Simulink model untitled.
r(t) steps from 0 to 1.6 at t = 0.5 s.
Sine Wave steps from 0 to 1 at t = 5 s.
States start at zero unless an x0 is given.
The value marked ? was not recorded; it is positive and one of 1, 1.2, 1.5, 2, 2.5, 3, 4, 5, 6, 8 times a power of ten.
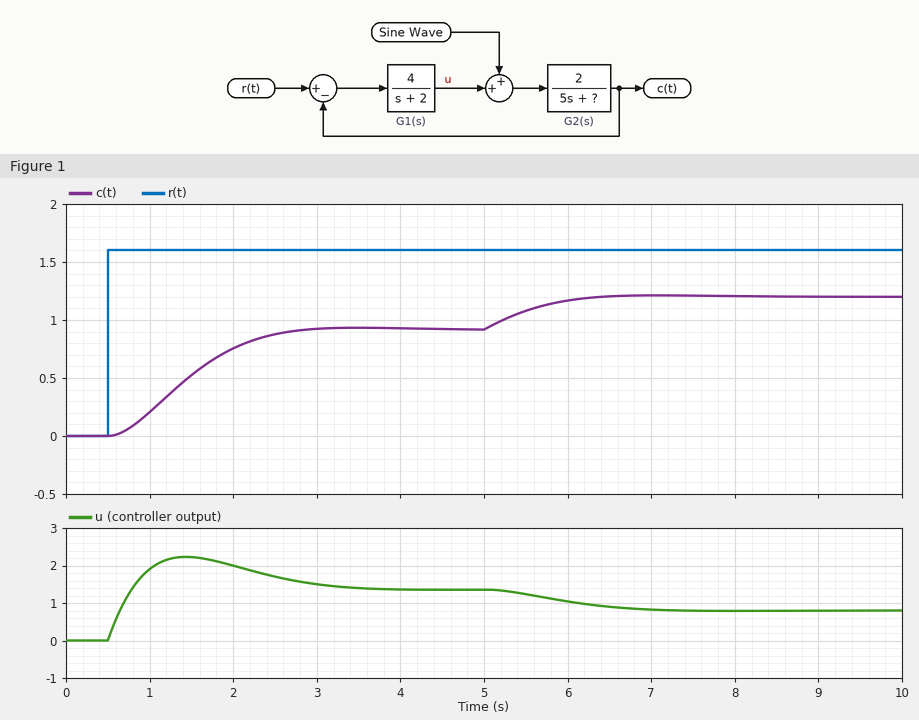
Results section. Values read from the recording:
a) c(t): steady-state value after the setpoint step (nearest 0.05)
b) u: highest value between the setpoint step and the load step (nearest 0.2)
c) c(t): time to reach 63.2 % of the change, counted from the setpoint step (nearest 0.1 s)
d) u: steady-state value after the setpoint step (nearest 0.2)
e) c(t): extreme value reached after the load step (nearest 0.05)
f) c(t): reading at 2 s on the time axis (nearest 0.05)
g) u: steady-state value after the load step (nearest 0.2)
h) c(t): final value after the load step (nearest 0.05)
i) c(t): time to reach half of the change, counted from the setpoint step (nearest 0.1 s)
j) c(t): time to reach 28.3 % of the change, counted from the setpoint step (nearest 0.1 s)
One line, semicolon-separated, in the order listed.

0.90; 2.2; 1.1 s; 1.4; 1.20; 0.75; 0.8; 1.20; 0.9 s; 0.6 s
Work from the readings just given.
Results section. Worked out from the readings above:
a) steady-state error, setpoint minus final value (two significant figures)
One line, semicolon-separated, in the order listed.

0.70
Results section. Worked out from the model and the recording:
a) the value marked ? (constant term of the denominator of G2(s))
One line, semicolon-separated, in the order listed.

3
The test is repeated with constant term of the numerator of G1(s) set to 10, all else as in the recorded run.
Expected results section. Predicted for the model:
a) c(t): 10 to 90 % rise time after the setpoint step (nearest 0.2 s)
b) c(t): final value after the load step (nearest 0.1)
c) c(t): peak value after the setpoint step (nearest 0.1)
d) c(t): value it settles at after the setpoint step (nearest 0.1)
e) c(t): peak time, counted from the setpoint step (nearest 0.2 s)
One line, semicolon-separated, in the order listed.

0.8 s; 1.4; 1.4; 1.2; 1.6 s
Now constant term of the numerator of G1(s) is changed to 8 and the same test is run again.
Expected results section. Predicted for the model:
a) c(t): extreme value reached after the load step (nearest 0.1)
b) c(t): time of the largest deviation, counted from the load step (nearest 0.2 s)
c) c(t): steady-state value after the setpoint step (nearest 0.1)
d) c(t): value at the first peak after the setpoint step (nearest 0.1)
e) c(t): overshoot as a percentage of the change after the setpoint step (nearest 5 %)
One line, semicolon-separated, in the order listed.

1.4; 1.2 s; 1.2; 1.3; 10 %
